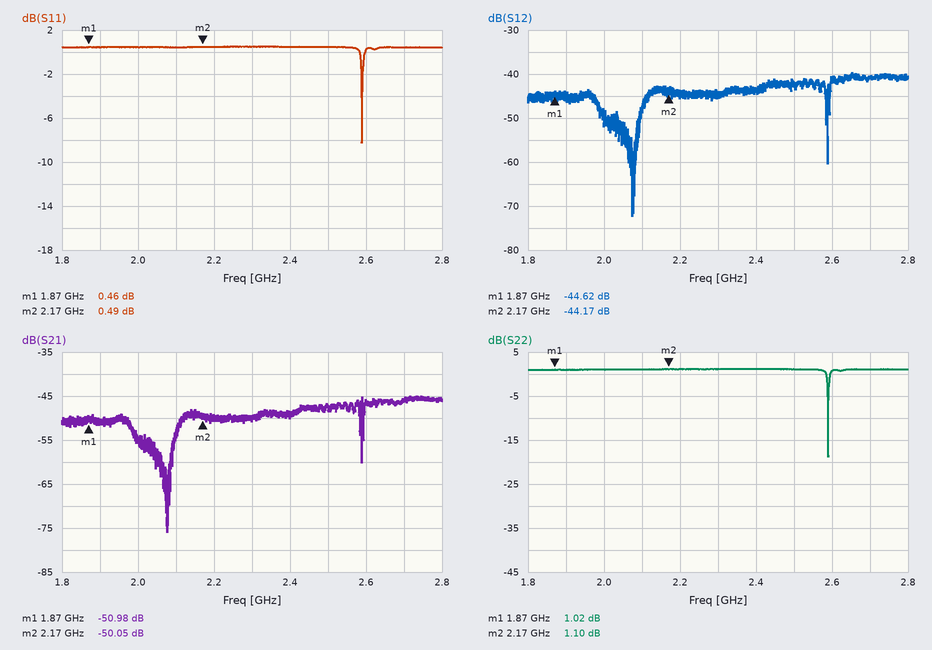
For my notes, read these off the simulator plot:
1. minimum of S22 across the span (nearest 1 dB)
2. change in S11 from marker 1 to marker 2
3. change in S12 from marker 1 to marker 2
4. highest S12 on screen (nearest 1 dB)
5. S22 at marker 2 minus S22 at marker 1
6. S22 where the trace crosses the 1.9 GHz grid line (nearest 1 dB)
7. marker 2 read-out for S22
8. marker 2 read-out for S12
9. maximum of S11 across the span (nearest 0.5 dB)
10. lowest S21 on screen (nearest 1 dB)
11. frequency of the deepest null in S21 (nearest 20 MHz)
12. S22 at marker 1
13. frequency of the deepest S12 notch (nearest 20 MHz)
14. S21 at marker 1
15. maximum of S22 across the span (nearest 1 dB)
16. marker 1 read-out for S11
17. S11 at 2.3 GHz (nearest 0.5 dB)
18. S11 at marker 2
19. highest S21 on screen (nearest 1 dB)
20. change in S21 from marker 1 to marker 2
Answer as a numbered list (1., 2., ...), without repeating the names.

1. -19 dB
2. 0.03 dB
3. 0.45 dB
4. -40 dB
5. 0.08 dB
6. 1 dB
7. 1.10 dB
8. -44.17 dB
9. 0.5 dB
10. -76 dB
11. 2.08 GHz
12. 1.02 dB
13. 2.08 GHz
14. -50.98 dB
15. 1 dB
16. 0.46 dB
17. 0.5 dB
18. 0.49 dB
19. -45 dB
20. 0.93 dB
